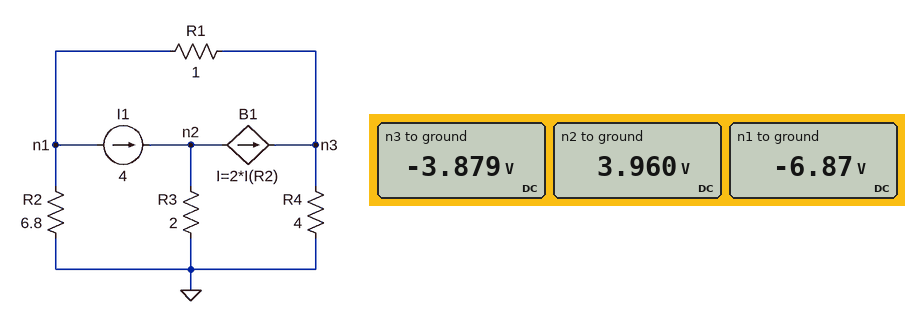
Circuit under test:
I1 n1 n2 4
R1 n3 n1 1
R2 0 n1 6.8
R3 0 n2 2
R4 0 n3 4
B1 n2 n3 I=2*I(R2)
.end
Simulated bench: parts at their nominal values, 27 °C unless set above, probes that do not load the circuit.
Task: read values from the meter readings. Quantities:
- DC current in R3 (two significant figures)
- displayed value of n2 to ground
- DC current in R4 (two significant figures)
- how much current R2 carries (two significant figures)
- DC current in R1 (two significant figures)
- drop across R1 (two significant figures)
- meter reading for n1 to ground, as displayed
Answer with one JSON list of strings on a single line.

["2.0 A", "3.960 V", "970 mA", "1.0 A", "3.0 A", "3.0 V", "-6.87 V"]
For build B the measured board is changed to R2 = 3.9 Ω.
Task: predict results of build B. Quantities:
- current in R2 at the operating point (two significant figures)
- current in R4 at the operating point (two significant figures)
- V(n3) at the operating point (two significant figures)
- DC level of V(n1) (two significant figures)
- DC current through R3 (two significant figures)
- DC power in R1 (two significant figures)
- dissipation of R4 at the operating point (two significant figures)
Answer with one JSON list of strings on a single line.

["1.2 A", "450 mA", "-1.8 V", "-4.6 V", "1.6 A", "7.9 W", "810 mW"]
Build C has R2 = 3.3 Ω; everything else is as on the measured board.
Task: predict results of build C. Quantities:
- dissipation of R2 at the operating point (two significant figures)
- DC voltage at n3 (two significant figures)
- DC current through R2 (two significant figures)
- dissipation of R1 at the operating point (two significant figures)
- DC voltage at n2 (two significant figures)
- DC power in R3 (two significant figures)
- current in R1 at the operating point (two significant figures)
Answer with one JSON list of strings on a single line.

["5.0 W", "-1.3 V", "1.2 A", "7.7 W", "3.1 V", "4.8 W", "2.8 A"]
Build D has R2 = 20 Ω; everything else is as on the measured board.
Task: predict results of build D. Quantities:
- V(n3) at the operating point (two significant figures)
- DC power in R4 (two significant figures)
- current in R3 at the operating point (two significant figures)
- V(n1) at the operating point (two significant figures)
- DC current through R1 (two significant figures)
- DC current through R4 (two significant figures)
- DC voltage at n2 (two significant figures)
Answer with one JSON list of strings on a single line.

["-8.7 V", "19 W", "2.8 A", "-12 V", "3.4 A", "2.2 A", "5.6 V"]
